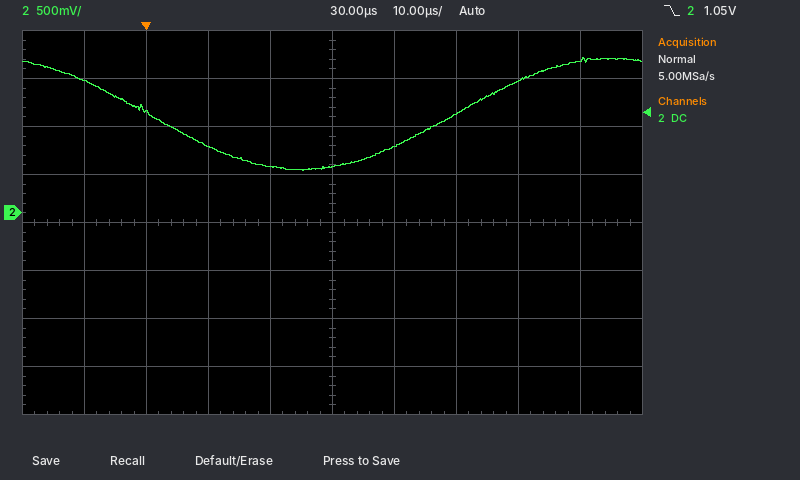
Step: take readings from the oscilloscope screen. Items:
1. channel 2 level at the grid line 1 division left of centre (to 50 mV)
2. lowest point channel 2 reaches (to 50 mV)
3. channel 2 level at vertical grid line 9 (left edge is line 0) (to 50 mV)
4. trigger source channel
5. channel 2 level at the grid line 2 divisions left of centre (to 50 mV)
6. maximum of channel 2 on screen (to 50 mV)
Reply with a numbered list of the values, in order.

1. 500 mV
2. 450 mV
3. 1.60 V
4. channel 2
5. 700 mV
6. 1.60 V
